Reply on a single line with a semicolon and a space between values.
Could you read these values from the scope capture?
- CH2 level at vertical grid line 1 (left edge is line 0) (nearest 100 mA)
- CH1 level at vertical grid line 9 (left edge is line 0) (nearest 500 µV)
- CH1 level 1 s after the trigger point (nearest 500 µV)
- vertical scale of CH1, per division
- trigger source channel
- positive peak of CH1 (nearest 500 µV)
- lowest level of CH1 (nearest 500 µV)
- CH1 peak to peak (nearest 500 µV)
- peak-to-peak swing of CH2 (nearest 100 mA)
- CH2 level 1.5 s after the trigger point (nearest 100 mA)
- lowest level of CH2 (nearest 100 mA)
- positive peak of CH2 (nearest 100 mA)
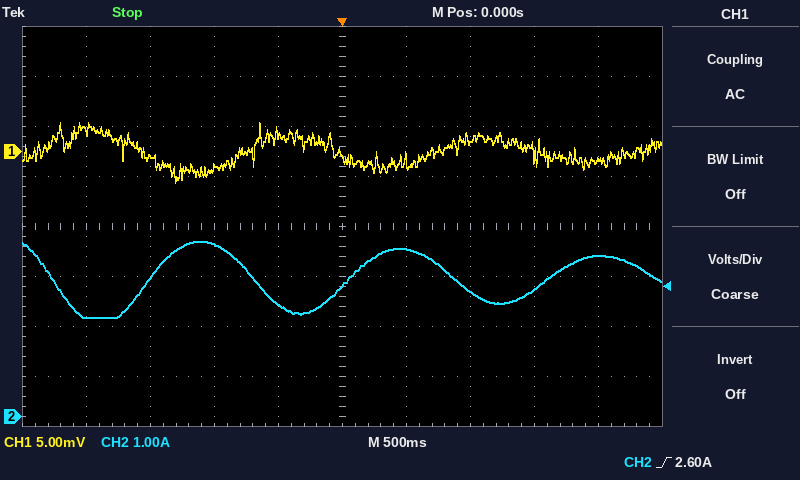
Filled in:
2.0 A; -1.0 mV; 1.0 mV; 5 mV; CH2; 3.0 mV; -3.0 mV; 6.0 mV; 1.5 A; 2.5 A; 2.0 A; 3.5 A
